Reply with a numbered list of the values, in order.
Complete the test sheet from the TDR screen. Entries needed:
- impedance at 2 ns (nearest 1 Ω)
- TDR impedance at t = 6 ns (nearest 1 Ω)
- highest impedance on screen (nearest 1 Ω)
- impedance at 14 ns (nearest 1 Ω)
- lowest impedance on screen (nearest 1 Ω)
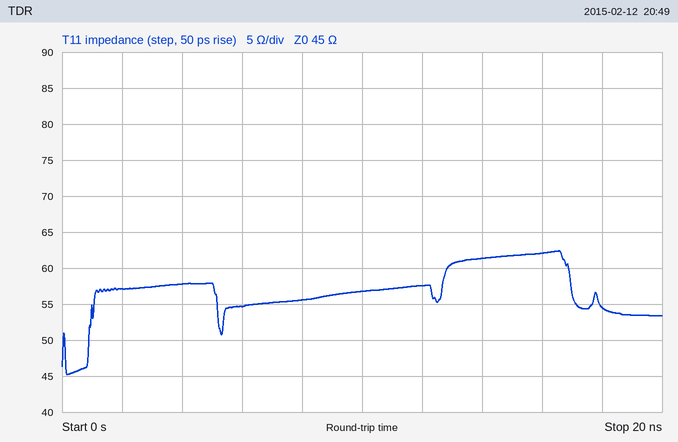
1. 57 Ω
2. 55 Ω
3. 62 Ω
4. 61 Ω
5. 45 Ω
